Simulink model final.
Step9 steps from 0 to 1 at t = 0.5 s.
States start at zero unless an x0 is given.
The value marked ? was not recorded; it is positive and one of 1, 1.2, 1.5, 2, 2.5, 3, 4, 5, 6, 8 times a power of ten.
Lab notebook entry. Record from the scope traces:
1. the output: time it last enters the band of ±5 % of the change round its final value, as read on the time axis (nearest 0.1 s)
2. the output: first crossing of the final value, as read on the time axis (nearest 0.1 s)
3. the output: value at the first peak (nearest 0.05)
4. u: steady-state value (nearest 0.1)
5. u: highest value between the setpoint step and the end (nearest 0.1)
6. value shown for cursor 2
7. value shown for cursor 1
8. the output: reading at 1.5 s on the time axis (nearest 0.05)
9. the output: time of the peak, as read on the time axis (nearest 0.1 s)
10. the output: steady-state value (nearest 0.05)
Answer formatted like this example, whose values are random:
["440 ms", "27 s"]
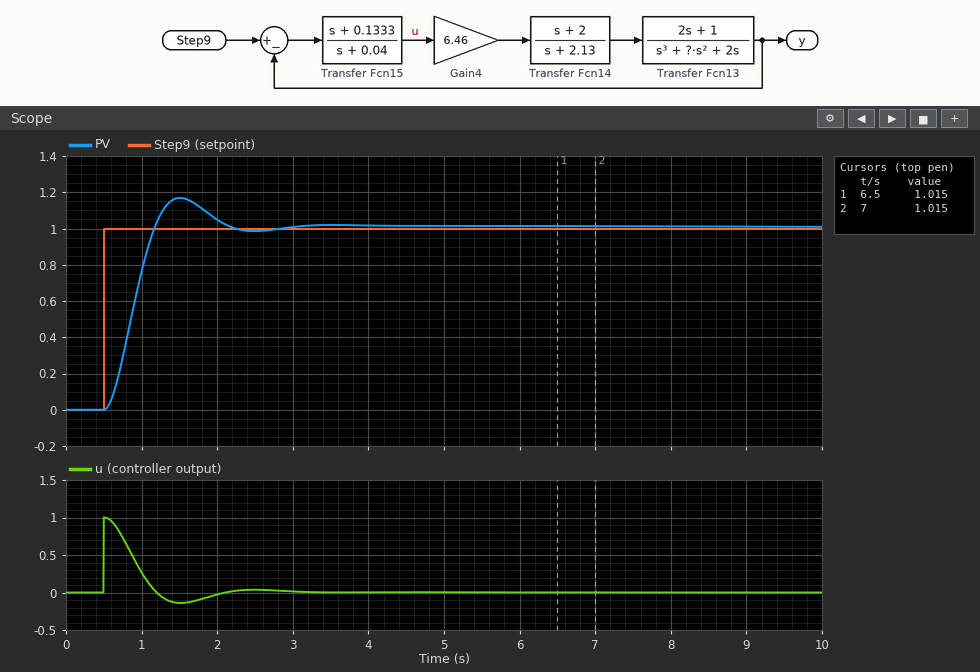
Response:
["2.0 s", "1.2 s", "1.15", "0.0", "1.0", "1.015", "1.015", "1.15", "1.5 s", "1.00"]
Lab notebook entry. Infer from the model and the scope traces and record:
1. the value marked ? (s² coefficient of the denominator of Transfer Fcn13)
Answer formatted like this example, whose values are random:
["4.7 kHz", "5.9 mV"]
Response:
["4"]
